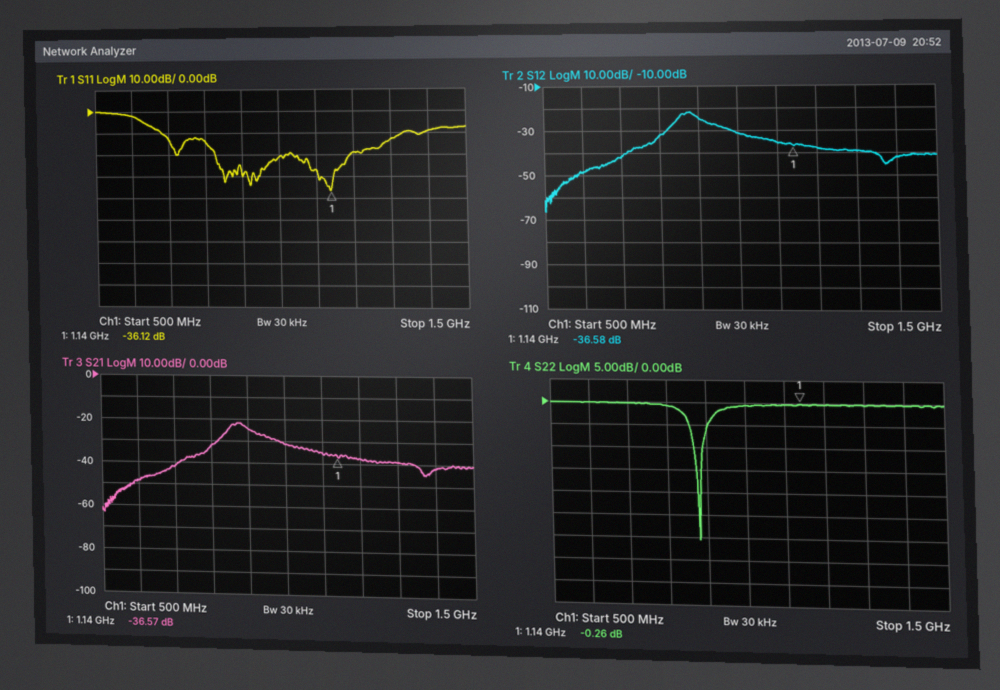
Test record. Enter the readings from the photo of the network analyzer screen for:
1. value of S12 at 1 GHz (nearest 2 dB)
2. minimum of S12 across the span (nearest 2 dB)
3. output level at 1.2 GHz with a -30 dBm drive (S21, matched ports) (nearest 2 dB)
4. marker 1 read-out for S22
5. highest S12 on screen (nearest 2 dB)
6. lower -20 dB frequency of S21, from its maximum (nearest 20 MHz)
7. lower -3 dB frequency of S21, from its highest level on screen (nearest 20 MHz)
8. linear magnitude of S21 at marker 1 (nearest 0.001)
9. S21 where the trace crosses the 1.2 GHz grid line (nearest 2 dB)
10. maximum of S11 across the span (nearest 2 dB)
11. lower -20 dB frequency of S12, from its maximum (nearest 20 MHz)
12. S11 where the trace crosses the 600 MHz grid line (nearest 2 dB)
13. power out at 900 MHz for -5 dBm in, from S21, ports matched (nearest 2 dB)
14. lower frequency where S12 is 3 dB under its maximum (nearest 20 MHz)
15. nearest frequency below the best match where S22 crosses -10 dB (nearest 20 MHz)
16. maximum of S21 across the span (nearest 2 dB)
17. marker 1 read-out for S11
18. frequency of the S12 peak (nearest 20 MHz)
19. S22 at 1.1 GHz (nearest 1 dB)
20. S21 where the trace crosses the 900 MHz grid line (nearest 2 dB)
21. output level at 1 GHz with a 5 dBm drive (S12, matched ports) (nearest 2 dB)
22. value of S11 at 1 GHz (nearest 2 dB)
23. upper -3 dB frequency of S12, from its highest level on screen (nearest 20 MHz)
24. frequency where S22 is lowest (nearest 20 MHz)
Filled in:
-32 dB
-66 dB
-68 dBm
-0.26 dB
-22 dB
700 MHz
840 MHz
0.015
-38 dB
0 dB
700 MHz
-2 dB
-30 dBm
840 MHz
860 MHz
-22 dB
-36.12 dB
880 MHz
0 dB
-24 dB
-26 dBm
-22 dB
900 MHz
880 MHz
